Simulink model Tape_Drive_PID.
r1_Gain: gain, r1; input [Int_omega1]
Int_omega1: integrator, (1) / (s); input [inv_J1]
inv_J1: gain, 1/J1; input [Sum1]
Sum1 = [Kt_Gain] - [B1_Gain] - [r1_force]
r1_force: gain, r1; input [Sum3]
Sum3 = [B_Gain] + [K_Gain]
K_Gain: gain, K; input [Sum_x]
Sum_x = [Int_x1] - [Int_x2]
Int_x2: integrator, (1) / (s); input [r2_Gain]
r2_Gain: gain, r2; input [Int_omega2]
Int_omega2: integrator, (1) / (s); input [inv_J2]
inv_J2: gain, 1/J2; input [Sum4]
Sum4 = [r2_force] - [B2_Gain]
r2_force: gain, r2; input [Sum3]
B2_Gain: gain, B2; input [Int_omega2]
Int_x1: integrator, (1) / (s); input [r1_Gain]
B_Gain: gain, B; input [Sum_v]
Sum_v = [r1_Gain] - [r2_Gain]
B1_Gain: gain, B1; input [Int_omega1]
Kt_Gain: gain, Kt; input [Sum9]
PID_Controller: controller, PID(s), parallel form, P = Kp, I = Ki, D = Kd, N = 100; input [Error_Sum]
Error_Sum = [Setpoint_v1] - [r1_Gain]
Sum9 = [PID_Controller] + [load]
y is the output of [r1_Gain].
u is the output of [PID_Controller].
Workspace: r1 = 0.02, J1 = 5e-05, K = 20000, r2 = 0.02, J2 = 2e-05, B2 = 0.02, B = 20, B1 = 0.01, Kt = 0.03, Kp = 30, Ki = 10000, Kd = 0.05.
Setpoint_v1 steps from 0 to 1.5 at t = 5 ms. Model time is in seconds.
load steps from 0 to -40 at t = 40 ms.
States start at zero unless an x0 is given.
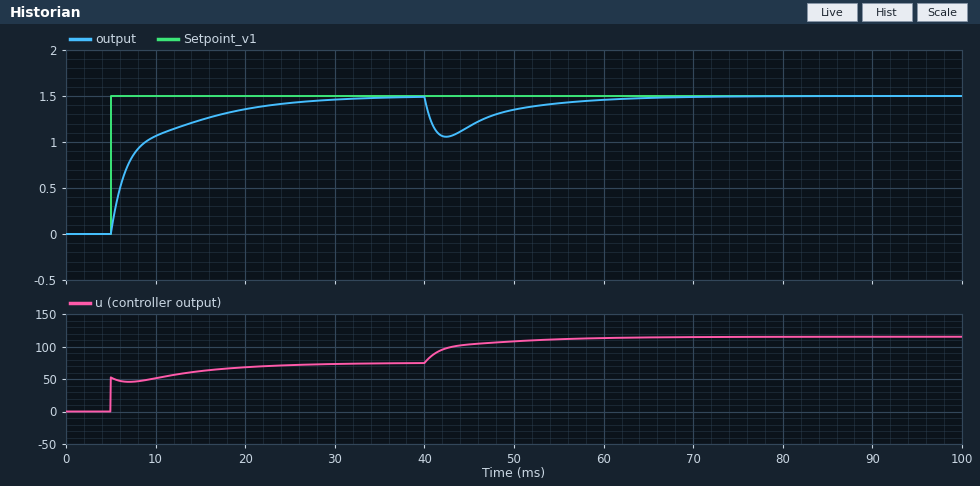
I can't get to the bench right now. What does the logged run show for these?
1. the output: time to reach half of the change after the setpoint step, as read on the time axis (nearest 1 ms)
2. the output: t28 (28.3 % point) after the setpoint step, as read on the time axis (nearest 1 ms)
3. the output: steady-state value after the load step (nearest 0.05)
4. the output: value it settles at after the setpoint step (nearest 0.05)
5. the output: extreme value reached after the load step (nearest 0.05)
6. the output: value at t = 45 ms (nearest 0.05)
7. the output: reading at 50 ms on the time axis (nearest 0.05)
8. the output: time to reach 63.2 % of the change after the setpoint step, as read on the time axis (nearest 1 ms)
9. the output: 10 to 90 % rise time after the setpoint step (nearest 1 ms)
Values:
7 ms
6 ms
1.50
1.50
1.05
1.15
1.35
8 ms
14 ms
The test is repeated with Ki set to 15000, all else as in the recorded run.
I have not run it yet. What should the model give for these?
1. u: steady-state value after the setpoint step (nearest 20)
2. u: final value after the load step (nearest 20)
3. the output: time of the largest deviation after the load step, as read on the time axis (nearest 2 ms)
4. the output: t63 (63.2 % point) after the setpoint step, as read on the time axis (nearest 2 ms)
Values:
80
120
42 ms
8 ms
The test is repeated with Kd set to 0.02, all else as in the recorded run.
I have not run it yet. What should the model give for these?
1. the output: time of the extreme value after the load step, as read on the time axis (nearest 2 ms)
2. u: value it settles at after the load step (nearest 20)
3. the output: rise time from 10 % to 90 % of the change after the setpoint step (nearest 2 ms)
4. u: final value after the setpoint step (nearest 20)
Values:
42 ms
120
14 ms
80
